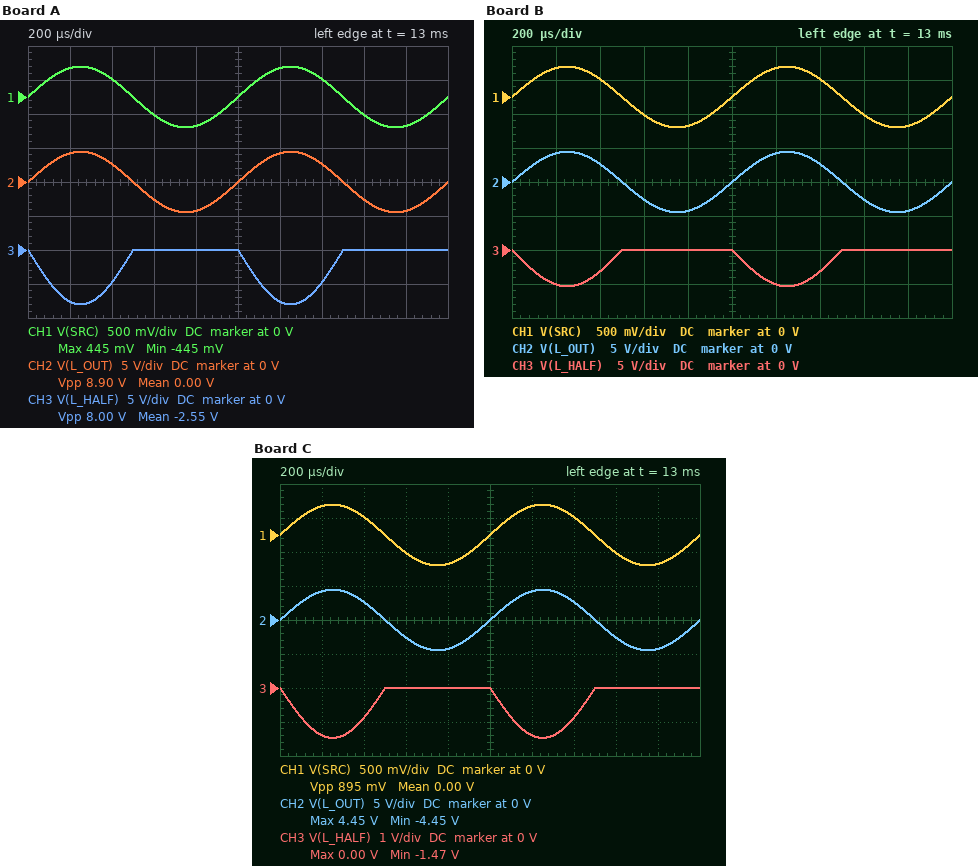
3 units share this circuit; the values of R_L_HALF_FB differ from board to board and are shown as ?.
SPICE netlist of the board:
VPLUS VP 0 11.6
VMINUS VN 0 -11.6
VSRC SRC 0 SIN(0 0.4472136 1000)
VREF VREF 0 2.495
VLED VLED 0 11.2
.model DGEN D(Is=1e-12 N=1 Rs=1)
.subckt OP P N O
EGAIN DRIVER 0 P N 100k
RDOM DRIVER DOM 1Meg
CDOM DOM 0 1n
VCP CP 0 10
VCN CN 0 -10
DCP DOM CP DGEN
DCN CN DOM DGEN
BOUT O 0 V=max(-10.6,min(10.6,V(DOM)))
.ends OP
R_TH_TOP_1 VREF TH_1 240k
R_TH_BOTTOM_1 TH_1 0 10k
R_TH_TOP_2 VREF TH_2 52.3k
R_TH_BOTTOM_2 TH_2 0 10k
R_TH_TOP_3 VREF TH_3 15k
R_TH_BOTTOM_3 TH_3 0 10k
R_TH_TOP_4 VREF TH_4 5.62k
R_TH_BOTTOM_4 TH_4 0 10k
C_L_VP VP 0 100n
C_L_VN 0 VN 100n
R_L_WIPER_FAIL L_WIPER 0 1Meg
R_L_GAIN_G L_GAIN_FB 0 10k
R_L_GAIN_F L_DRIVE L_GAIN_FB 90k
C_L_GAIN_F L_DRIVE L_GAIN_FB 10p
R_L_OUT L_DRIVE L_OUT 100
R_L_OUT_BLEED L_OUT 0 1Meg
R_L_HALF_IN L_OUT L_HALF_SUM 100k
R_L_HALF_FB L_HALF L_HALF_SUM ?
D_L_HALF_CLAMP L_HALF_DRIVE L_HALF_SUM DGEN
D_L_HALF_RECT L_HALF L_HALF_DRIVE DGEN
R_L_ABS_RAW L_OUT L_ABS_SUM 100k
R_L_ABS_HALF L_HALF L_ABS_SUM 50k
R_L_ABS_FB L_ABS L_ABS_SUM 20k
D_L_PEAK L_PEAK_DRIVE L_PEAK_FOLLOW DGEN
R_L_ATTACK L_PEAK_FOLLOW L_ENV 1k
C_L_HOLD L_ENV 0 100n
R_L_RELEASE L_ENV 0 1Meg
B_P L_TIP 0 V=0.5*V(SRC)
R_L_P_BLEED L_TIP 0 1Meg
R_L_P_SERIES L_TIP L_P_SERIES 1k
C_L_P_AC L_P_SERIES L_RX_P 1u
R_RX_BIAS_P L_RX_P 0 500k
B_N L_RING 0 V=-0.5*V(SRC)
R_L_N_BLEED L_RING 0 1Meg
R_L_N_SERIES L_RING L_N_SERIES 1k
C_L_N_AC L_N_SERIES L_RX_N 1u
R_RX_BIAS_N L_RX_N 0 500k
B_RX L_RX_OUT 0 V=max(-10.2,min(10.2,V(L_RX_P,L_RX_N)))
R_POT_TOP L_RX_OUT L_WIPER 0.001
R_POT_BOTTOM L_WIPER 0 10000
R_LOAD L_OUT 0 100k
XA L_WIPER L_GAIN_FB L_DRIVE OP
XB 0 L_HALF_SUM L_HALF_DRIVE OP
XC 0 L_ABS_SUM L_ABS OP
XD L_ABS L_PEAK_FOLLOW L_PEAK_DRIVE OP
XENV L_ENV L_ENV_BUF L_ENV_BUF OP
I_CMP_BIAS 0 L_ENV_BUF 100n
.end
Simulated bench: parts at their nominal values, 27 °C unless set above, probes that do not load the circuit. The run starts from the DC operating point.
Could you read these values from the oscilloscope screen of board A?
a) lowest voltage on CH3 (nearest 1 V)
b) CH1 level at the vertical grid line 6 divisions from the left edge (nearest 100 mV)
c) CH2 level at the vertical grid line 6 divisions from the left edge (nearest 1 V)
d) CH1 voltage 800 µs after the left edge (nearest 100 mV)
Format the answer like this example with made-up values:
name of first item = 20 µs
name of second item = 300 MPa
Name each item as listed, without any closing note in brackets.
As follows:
lowest voltage on CH3 = -8 V
CH1 level at the vertical grid line 6 divisions from the left edge = 400 mV
CH2 level at the vertical grid line 6 divisions from the left edge = 4 V
CH1 voltage 800 µs after the left edge = -400 mV
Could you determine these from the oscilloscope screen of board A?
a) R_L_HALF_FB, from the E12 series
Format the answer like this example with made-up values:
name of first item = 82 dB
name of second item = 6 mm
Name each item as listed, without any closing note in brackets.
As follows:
R_L_HALF_FB, from the E12 series = 180 kΩ
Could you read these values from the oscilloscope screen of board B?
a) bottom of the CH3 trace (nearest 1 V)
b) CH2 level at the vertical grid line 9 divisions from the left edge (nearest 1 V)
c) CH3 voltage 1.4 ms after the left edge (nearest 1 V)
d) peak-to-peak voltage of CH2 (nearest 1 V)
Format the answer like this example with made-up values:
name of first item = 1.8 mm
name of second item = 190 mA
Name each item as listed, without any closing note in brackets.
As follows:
bottom of the CH3 trace = -5 V
CH2 level at the vertical grid line 9 divisions from the left edge = -4 V
CH3 voltage 1.4 ms after the left edge = -3 V
peak-to-peak voltage of CH2 = 9 V
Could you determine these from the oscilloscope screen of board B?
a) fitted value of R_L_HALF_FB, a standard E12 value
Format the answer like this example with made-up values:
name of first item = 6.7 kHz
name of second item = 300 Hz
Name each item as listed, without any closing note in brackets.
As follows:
fitted value of R_L_HALF_FB, a standard E12 value = 120 kΩ
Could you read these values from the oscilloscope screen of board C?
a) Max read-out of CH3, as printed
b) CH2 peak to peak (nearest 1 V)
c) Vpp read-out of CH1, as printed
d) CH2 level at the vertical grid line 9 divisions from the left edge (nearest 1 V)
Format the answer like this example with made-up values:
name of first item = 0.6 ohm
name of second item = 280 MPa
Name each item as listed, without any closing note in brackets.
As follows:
Max read-out of CH3, as printed = 0.00 V
CH2 peak to peak = 9 V
Vpp read-out of CH1, as printed = 895 mV
CH2 level at the vertical grid line 9 divisions from the left edge = -4 V
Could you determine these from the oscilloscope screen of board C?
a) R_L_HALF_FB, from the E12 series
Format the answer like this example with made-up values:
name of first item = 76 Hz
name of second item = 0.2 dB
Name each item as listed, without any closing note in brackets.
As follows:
R_L_HALF_FB, from the E12 series = 33 kΩ
